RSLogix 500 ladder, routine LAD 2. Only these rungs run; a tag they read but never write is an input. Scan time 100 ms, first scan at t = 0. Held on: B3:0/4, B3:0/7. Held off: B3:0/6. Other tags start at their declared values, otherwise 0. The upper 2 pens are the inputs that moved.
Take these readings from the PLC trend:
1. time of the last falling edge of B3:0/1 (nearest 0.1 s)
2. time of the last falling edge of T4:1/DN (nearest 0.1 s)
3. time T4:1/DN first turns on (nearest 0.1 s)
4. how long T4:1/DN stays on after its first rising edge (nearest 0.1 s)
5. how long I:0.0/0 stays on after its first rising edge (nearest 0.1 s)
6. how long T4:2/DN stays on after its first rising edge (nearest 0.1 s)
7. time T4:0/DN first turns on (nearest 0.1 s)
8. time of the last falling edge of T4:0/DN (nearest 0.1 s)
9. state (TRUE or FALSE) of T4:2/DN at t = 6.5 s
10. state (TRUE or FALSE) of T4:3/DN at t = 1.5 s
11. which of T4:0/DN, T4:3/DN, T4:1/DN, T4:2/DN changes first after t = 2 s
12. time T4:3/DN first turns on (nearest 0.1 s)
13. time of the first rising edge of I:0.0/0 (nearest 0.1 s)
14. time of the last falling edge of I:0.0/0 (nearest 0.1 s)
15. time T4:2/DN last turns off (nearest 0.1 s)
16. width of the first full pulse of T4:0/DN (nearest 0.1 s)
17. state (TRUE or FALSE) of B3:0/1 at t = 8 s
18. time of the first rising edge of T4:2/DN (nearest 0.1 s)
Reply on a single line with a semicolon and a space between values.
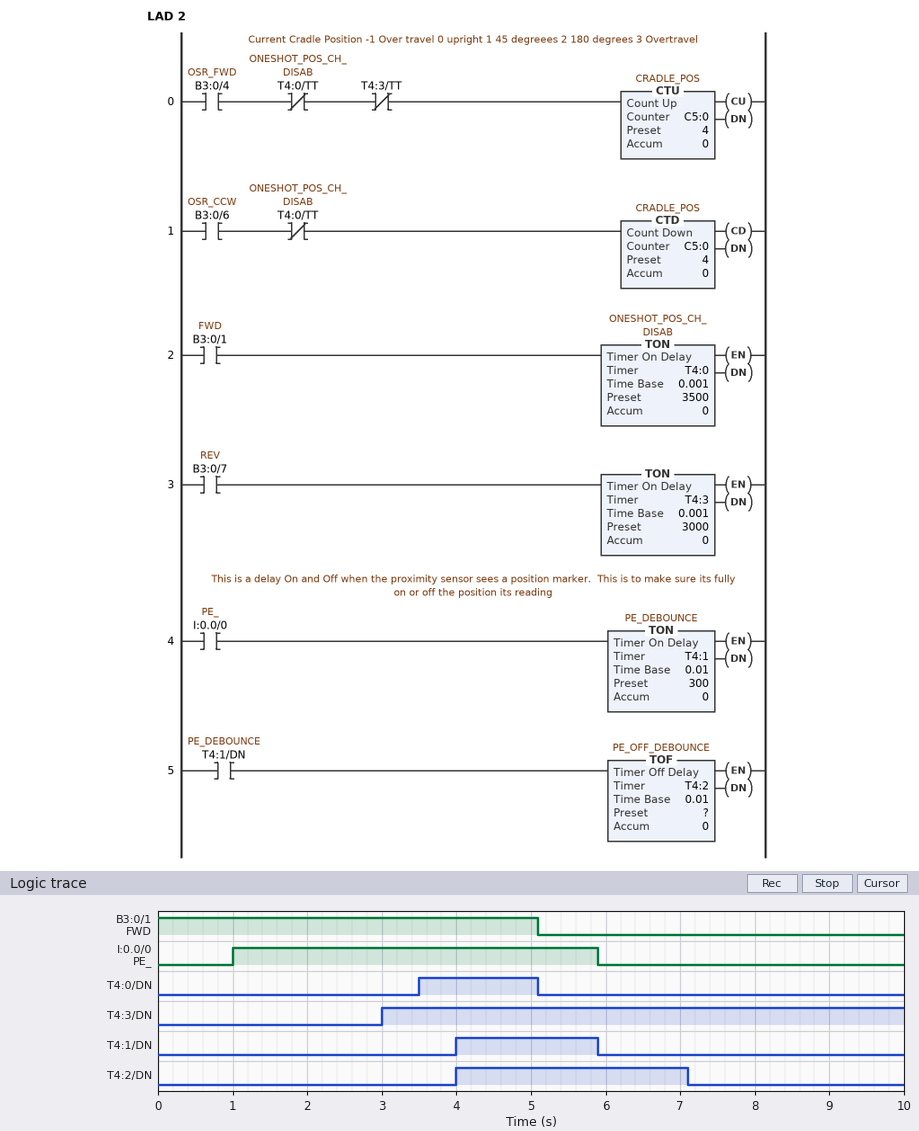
5.1 s; 5.9 s; 4.0 s; 1.9 s; 4.9 s; 3.1 s; 3.5 s; 5.1 s; TRUE; FALSE; T4:3/DN; 3.0 s; 1.0 s; 5.9 s; 7.1 s; 1.6 s; FALSE; 4.0 s
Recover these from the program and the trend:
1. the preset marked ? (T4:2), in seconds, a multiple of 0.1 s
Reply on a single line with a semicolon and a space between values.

1.2 s
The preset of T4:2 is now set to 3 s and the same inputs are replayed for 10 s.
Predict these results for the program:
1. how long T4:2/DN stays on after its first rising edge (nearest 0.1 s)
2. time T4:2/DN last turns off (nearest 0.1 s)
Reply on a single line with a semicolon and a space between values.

4.9 s; 8.9 s
